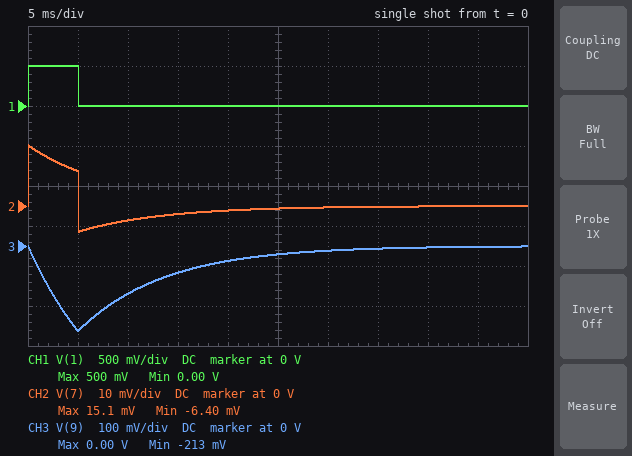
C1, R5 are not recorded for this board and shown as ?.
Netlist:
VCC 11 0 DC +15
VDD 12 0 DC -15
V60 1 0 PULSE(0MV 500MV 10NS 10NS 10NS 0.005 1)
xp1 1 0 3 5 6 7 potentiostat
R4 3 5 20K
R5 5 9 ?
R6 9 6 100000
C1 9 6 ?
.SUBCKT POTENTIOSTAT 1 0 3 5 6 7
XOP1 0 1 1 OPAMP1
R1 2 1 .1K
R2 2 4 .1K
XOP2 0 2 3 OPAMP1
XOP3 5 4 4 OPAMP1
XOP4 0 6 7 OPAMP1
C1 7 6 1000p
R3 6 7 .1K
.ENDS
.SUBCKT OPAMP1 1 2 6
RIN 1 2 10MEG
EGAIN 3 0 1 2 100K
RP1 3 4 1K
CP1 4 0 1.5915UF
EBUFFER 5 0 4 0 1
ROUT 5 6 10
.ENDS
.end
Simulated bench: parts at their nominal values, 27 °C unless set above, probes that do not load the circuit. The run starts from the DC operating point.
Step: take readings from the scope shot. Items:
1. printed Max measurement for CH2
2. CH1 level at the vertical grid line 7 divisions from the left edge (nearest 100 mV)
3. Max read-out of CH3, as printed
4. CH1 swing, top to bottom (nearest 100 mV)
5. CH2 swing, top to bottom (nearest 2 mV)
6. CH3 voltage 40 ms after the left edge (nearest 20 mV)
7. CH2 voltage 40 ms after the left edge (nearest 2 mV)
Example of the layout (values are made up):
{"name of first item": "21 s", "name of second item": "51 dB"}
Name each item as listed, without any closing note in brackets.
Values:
{"printed Max measurement for CH2": "15.1 mV", "CH1 level at the vertical grid line 7 divisions from the left edge": "0 V", "Max read-out of CH3, as printed": "0.00 V", "CH1 swing, top to bottom": "500 mV", "CH2 swing, top to bottom": "22 mV", "CH3 voltage 40 ms after the left edge": "0 V", "CH2 voltage 40 ms after the left edge": "0 V"}
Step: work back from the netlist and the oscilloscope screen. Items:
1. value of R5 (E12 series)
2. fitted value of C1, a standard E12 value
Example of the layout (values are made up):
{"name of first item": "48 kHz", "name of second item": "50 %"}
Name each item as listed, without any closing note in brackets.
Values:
{"value of R5": "3.3 kΩ", "fitted value of C1, a standard E12 value": "2.7 µF"}
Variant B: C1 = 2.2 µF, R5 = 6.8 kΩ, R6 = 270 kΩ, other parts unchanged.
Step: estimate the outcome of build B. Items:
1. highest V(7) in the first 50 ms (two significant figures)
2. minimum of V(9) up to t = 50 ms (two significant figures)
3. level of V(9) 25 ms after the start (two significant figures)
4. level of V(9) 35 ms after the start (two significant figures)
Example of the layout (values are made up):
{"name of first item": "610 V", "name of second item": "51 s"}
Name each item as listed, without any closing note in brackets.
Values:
{"highest V(7) in the first 50 ms": "7.4 mV", "minimum of V(9) up to t = 50 ms": "-140 mV", "level of V(9) 25 ms after the start": "-36 mV", "level of V(9) 35 ms after the start": "-18 mV"}
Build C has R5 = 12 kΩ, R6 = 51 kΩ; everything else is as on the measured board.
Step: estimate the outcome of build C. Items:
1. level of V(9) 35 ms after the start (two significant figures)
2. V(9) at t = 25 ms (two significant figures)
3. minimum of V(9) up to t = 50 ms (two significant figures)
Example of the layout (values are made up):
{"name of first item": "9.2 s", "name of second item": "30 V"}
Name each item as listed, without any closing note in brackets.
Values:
{"level of V(9) 35 ms after the start": "-22 mV", "V(9) at t = 25 ms": "-33 mV", "minimum of V(9) up to t = 50 ms": "-70 mV"}
